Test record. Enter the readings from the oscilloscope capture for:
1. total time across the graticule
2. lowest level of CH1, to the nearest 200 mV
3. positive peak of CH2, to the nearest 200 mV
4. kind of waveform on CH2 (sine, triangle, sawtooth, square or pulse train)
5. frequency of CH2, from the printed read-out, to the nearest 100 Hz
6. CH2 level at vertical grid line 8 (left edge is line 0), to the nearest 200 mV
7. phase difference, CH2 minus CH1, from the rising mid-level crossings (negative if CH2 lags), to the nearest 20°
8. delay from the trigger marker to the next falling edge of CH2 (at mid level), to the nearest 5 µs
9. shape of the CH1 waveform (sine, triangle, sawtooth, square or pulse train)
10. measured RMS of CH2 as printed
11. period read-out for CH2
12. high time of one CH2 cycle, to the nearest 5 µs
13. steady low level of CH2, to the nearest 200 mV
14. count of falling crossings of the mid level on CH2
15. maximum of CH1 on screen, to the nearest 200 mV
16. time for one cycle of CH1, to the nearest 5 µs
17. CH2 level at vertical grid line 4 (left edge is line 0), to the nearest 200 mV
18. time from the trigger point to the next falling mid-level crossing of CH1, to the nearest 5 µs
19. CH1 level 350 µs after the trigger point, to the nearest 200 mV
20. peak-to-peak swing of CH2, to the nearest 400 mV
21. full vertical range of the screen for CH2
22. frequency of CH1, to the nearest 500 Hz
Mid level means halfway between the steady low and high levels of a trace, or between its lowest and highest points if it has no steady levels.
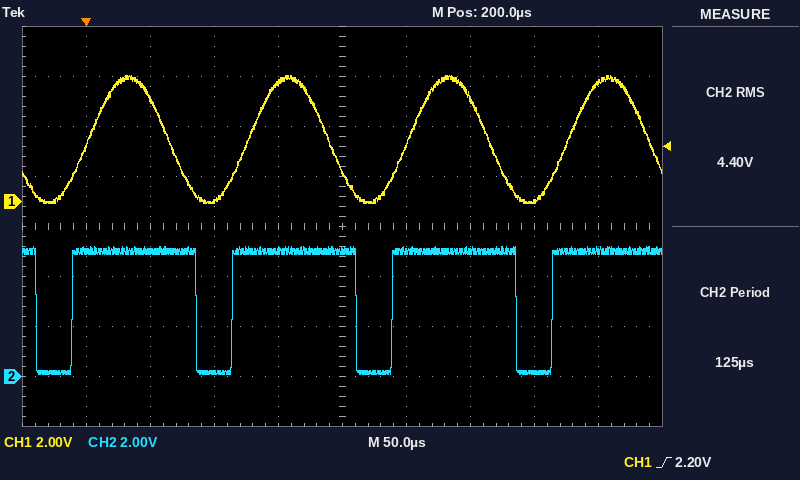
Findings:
500 µs
0.0 V
5.2 V
pulse train
8.0 kHz
200 mV
+40°
85 µs
sine
4.40 V
125 µs
95 µs
200 mV
4
5.0 V
125 µs
5.0 V
65 µs
0.0 V
5.2 V
16 V
8.0 kHz
